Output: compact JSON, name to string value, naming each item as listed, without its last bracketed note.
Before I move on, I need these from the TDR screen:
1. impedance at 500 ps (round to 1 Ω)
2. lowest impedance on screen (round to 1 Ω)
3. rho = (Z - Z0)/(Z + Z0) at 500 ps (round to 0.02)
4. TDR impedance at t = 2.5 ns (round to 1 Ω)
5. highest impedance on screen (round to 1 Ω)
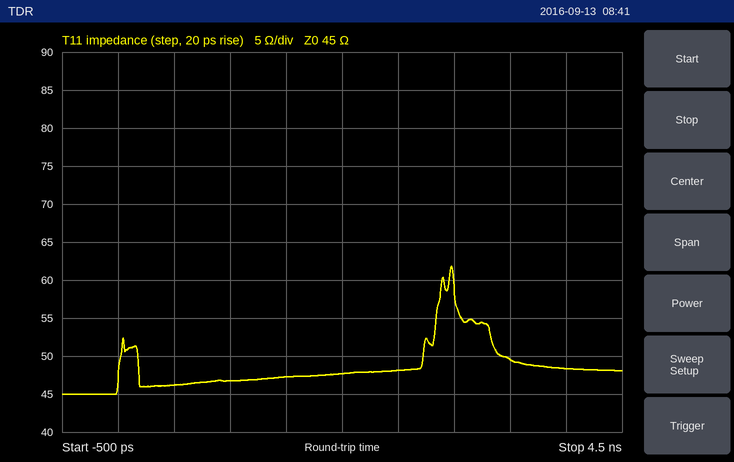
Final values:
{"impedance at 500 ps": "46 Ω", "lowest impedance on screen": "45 Ω", "rho = (Z - Z0)/(Z + Z0) at 500 ps": "+0.02", "TDR impedance at t = 2.5 ns": "48 Ω", "highest impedance on screen": "62 Ω"}
